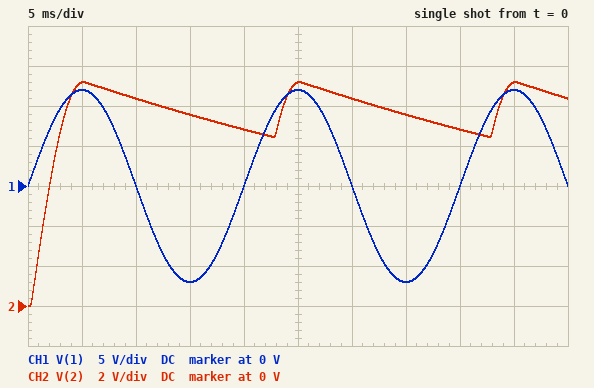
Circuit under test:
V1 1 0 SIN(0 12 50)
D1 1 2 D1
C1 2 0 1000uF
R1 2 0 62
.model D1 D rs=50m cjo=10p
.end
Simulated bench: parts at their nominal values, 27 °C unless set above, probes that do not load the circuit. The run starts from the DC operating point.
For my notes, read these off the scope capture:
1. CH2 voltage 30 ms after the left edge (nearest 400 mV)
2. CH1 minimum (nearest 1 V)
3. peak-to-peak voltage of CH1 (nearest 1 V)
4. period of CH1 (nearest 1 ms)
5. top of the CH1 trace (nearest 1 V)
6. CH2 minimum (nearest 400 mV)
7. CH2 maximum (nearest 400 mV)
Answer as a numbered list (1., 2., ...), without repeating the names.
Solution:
1. 10.4 V
2. -12 V
3. 24 V
4. 20 ms
5. 12 V
6. 0 V
7. 11.2 V
